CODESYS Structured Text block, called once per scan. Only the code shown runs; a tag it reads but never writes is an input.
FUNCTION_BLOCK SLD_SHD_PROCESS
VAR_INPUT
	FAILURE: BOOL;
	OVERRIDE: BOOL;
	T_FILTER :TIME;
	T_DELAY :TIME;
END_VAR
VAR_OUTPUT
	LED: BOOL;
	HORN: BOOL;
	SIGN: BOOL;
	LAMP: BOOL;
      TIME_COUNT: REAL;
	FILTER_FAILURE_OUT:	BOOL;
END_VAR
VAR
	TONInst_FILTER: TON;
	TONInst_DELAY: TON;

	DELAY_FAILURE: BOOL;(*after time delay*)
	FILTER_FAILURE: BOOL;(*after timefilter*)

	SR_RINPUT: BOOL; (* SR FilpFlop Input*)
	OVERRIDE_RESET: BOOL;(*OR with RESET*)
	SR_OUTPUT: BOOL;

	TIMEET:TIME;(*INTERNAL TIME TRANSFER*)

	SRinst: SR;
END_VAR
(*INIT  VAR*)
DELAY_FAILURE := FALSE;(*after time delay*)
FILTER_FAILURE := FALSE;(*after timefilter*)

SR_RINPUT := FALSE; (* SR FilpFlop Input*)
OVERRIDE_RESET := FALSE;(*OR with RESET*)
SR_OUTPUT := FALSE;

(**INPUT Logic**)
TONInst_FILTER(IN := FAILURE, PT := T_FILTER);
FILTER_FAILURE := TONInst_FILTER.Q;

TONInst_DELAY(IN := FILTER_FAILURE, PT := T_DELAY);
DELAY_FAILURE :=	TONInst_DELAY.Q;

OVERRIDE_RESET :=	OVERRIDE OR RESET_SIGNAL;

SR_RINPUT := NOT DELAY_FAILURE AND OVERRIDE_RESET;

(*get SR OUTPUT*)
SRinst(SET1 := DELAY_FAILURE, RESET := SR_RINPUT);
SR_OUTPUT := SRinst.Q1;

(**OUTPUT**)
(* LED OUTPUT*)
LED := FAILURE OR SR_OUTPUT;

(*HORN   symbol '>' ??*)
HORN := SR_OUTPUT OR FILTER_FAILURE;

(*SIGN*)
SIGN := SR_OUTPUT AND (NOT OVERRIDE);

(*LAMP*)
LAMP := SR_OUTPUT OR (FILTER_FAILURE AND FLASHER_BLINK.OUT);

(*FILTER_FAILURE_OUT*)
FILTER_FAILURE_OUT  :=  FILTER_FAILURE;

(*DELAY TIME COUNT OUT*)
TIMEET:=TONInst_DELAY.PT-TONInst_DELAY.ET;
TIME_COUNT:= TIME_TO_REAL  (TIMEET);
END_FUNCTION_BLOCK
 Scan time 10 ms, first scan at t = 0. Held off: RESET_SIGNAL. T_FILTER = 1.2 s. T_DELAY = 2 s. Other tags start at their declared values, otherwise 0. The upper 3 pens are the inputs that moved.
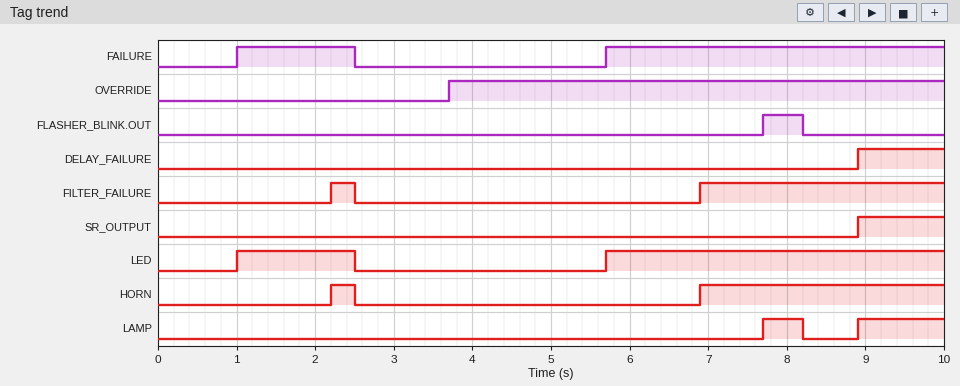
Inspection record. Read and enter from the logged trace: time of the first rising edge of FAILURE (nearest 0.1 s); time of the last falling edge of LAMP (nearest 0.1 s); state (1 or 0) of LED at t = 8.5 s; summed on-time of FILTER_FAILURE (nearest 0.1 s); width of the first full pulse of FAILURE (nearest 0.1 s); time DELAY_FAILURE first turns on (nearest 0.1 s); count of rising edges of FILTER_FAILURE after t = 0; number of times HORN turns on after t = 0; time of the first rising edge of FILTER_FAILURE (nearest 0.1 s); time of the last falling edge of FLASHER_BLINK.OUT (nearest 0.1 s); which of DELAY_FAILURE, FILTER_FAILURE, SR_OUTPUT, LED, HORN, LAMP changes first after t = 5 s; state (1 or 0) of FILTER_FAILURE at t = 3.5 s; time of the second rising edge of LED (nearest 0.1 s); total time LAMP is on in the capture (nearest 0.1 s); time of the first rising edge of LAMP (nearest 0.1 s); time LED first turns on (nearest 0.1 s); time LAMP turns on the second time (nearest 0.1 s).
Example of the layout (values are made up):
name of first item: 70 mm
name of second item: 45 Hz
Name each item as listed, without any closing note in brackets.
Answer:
time of the first rising edge of FAILURE: 1.0 s
time of the last falling edge of LAMP: 8.2 s
state (1 or 0) of LED at t = 8.5 s: 1
summed on-time of FILTER_FAILURE: 3.4 s
width of the first full pulse of FAILURE: 1.5 s
time DELAY_FAILURE first turns on: 8.9 s
count of rising edges of FILTER_FAILURE after t = 0: 2
number of times HORN turns on after t = 0: 2
time of the first rising edge of FILTER_FAILURE: 2.2 s
time of the last falling edge of FLASHER_BLINK.OUT: 8.2 s
which of DELAY_FAILURE, FILTER_FAILURE, SR_OUTPUT, LED, HORN, LAMP changes first after t = 5 s: LED
state (1 or 0) of FILTER_FAILURE at t = 3.5 s: 0
time of the second rising edge of LED: 5.7 s
total time LAMP is on in the capture: 1.6 s
time of the first rising edge of LAMP: 7.7 s
time LED first turns on: 1.0 s
time LAMP turns on the second time: 8.9 s
